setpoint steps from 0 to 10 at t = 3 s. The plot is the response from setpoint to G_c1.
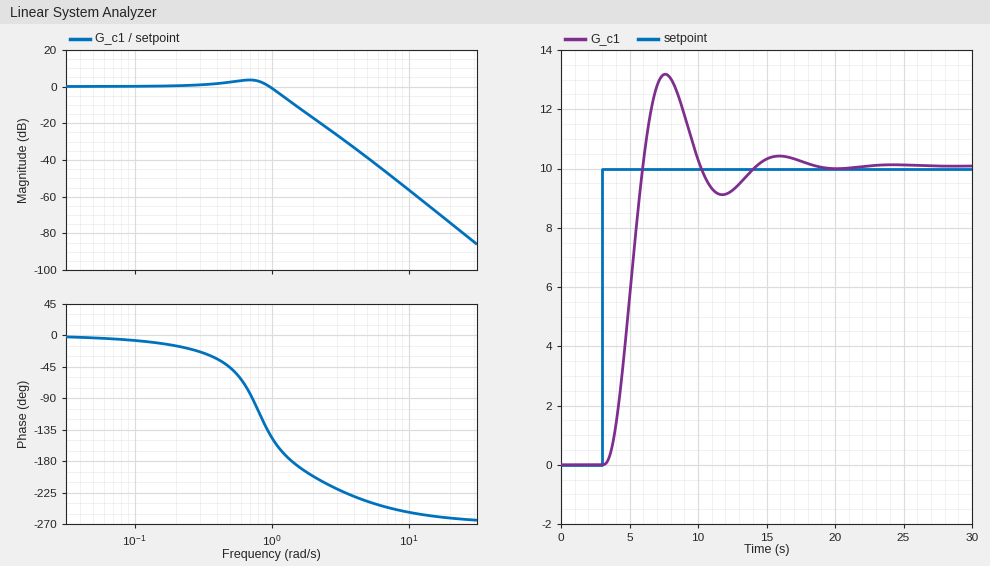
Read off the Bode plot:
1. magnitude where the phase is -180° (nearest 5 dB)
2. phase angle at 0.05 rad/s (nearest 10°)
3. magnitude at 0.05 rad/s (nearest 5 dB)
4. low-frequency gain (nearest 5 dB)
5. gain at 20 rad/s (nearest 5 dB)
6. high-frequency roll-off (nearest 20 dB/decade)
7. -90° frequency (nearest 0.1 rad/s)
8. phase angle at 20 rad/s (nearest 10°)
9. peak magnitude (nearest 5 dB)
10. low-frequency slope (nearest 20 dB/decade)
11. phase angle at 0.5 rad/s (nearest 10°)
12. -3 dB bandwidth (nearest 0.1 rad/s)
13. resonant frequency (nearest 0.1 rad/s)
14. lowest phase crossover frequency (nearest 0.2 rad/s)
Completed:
-10 dB
0°
0 dB
0 dB
-75 dB
-60 dB/decade
0.7 rad/s
-260°
5 dB
0 dB/decade
-50°
1.1 rad/s
0.7 rad/s
1.4 rad/s
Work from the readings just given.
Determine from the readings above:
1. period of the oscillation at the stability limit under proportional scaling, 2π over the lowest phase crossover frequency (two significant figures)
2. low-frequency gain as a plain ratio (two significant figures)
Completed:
4.5 s
1.0
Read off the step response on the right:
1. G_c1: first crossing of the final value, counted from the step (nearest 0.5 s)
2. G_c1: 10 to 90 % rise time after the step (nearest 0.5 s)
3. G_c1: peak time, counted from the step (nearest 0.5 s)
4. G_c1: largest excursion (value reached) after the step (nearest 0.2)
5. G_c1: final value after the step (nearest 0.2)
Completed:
3.0 s
2.0 s
4.5 s
13.2
10.0
